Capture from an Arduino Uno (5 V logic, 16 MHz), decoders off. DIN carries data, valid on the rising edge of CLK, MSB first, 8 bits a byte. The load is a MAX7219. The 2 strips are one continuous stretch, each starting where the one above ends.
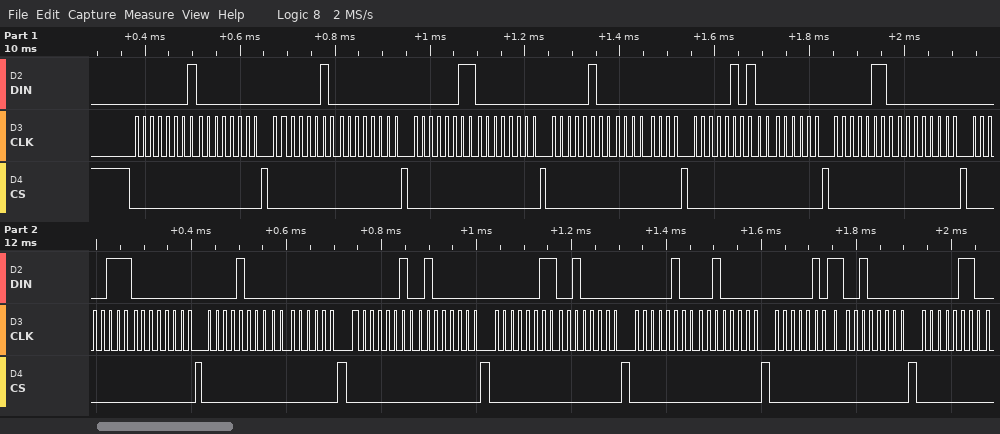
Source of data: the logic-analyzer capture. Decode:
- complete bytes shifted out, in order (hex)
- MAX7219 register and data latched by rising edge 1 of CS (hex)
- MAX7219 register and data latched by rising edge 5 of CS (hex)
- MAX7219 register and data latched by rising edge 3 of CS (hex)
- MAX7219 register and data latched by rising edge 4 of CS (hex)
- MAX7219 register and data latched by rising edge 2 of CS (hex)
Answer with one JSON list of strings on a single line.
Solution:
["01 00 02 00 03 00 04 00 05 00 06 00 07 00 08 00 02 40 03 20 04 20 05 20 06", "register 0x1, data 0x00", "register 0x5, data 0x00", "register 0x3, data 0x00", "register 0x4, data 0x00", "register 0x2, data 0x00"]
